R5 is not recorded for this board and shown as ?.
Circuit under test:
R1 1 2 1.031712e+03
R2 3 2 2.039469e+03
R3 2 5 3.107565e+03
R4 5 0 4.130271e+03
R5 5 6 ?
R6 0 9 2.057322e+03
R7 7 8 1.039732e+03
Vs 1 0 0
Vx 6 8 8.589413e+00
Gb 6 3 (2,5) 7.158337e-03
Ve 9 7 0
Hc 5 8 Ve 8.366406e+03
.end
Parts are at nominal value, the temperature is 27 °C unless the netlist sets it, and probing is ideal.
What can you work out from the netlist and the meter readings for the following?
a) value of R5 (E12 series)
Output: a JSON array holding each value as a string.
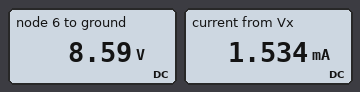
["5.6 kΩ"]
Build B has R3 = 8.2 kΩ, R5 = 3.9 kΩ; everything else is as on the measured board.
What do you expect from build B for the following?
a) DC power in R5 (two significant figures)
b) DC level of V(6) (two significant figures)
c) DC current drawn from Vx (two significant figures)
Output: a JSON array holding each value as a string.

["19 mW", "8.6 V", "2.2 mA"]
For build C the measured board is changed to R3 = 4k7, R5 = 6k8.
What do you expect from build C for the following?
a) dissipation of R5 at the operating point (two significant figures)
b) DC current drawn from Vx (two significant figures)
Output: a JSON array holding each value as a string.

["11 mW", "1.3 mA"]
